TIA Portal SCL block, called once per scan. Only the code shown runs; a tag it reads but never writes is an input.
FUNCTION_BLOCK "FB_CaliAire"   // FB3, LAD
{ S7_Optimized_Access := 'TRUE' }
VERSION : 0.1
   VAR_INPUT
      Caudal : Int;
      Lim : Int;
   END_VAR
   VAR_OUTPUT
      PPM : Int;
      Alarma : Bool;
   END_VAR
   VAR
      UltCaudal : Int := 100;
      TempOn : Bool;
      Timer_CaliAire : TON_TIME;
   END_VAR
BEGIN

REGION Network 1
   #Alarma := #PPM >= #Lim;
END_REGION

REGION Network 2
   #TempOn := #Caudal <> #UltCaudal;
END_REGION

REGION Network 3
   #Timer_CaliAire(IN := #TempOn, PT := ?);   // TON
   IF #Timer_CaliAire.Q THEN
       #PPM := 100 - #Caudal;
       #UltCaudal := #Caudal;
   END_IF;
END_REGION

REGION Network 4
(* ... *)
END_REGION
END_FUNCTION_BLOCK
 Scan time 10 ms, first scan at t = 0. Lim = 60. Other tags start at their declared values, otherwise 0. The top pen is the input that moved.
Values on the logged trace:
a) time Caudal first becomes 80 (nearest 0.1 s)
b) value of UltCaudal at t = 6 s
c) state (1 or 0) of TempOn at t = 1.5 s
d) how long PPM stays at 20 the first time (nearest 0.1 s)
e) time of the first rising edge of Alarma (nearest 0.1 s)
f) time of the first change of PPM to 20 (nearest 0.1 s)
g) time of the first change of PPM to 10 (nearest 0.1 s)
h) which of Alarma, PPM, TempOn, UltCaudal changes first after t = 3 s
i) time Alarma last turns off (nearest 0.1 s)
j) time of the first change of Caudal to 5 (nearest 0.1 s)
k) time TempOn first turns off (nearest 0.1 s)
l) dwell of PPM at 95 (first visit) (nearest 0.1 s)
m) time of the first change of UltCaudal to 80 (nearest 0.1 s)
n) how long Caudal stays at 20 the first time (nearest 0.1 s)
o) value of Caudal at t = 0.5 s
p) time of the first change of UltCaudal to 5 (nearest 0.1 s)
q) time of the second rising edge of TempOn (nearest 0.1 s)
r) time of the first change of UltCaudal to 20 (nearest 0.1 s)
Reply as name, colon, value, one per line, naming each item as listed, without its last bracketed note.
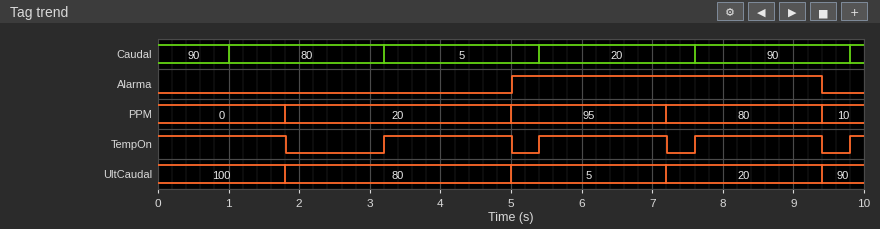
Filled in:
time Caudal first becomes 80: 1.0 s
value of UltCaudal at t = 6 s: 5
state (1 or 0) of TempOn at t = 1.5 s: 1
how long PPM stays at 20 the first time: 3.2 s
time of the first rising edge of Alarma: 5.0 s
time of the first change of PPM to 20: 1.8 s
time of the first change of PPM to 10: 9.4 s
which of Alarma, PPM, TempOn, UltCaudal changes first after t = 3 s: TempOn
time Alarma last turns off: 9.4 s
time of the first change of Caudal to 5: 3.2 s
time TempOn first turns off: 1.8 s
dwell of PPM at 95 (first visit): 2.2 s
time of the first change of UltCaudal to 80: 1.8 s
how long Caudal stays at 20 the first time: 2.2 s
value of Caudal at t = 0.5 s: 90
time of the first change of UltCaudal to 5: 5.0 s
time of the second rising edge of TempOn: 5.4 s
time of the first change of UltCaudal to 20: 7.2 s
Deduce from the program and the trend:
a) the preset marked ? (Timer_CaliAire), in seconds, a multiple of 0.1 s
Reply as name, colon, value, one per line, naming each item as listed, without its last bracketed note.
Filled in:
the preset marked ? (Timer_CaliAire), in seconds, a multiple of 0.1 s: 1.8 s
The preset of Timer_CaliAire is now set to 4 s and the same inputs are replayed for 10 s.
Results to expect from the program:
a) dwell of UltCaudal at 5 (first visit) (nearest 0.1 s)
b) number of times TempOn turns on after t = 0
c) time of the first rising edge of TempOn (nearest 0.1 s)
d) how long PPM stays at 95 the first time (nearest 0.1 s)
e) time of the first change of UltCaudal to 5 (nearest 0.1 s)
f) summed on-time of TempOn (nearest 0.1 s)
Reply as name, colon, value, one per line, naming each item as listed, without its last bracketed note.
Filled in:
dwell of UltCaudal at 5 (first visit): 5.4 s
number of times TempOn turns on after t = 0: 2
time of the first rising edge of TempOn: 5.4 s
how long PPM stays at 95 the first time: 5.4 s
time of the first change of UltCaudal to 5: 4.0 s
summed on-time of TempOn: 8.2 s
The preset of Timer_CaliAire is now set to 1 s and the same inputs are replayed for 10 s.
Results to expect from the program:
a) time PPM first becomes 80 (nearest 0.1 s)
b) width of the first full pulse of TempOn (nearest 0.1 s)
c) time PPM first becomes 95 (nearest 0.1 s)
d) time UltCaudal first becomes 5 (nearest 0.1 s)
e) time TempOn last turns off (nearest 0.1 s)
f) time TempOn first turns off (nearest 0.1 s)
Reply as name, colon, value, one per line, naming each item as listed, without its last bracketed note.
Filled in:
time PPM first becomes 80: 6.4 s
width of the first full pulse of TempOn: 1.0 s
time PPM first becomes 95: 4.2 s
time UltCaudal first becomes 5: 4.2 s
time TempOn last turns off: 8.6 s
time TempOn first turns off: 1.0 s
